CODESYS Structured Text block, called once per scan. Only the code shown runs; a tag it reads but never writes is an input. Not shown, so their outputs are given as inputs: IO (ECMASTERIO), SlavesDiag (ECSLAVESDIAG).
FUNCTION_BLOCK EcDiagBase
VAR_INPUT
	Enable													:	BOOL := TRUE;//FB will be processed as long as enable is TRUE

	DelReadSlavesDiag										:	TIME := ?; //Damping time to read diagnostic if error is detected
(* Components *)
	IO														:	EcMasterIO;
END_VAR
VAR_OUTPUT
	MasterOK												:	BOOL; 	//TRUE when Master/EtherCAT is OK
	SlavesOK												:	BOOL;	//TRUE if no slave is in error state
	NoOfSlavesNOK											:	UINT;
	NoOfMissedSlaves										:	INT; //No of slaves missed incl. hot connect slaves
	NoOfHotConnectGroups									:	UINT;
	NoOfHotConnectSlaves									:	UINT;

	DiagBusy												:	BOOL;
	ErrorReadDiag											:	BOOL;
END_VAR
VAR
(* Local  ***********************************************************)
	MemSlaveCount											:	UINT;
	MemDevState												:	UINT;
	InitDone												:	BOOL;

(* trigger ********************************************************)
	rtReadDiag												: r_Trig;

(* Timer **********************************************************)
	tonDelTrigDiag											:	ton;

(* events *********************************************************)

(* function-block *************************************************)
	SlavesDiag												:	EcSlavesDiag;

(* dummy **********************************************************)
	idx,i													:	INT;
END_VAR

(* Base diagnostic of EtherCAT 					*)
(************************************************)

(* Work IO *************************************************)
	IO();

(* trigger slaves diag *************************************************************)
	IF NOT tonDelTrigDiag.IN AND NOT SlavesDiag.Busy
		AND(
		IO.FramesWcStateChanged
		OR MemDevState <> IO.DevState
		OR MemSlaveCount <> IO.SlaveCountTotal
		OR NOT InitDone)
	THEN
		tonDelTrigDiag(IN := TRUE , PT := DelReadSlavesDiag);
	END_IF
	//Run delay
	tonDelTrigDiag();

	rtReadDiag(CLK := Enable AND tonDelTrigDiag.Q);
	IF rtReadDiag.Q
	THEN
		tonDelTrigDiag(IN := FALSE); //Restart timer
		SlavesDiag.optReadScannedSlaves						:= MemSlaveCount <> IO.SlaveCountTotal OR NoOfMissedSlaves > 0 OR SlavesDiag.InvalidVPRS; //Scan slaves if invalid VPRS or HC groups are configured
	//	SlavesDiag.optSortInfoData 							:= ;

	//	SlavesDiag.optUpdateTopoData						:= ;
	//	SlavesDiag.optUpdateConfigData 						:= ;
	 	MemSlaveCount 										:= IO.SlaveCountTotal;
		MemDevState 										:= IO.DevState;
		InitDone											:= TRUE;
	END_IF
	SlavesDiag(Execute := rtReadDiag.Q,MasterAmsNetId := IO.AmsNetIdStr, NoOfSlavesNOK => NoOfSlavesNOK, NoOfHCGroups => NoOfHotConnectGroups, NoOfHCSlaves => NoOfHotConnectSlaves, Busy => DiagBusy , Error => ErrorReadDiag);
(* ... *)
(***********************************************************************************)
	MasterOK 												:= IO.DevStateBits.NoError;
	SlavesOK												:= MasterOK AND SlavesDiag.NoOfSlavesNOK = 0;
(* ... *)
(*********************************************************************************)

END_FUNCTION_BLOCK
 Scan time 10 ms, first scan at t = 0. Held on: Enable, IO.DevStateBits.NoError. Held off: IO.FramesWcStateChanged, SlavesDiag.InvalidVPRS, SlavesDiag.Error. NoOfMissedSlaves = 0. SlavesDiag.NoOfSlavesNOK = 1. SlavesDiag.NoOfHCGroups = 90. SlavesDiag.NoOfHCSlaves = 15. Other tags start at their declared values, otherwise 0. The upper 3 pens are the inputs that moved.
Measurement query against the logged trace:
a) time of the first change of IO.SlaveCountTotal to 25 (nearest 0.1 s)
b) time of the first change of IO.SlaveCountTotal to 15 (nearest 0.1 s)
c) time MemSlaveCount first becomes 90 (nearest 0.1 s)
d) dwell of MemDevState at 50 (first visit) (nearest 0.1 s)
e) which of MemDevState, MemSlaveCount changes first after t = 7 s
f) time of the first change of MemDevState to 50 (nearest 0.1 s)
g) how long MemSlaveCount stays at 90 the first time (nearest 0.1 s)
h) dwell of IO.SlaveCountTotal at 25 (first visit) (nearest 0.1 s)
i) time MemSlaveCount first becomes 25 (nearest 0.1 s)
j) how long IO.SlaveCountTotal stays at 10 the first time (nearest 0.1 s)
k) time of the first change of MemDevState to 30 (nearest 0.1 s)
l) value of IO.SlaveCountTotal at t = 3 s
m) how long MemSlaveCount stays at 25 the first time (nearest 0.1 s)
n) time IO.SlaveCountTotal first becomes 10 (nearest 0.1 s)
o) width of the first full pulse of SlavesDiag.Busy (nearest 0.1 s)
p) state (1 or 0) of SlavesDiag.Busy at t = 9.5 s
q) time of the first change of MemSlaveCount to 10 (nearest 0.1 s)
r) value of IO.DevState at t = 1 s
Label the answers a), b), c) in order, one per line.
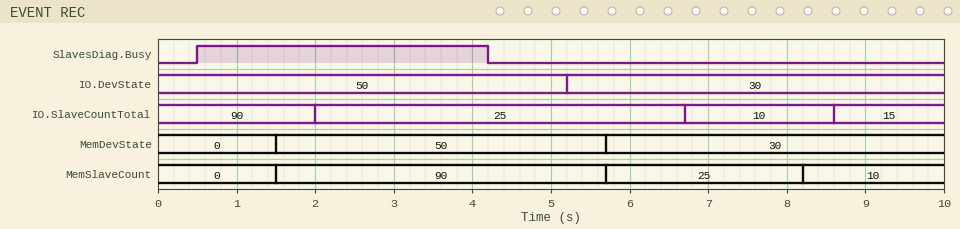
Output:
a) 2.0 s
b) 8.6 s
c) 1.5 s
d) 4.2 s
e) MemSlaveCount
f) 1.5 s
g) 4.2 s
h) 4.7 s
i) 5.7 s
j) 1.9 s
k) 5.7 s
l) 25
m) 2.5 s
n) 6.7 s
o) 3.7 s
p) 0
q) 8.2 s
r) 50
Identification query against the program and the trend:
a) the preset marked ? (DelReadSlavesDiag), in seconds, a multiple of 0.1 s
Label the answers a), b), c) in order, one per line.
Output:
a) 1.5 s
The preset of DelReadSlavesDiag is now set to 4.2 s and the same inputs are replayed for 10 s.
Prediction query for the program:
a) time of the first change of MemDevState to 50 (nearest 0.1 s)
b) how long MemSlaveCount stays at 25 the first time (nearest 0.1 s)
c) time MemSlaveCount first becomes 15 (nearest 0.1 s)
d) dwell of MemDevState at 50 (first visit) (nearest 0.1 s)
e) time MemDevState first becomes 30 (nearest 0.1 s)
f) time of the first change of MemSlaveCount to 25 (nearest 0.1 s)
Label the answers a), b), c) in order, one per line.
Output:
a) 4.2 s
b) 5.2 s
c) 9.4 s
d) 5.2 s
e) 9.4 s
f) 4.2 s
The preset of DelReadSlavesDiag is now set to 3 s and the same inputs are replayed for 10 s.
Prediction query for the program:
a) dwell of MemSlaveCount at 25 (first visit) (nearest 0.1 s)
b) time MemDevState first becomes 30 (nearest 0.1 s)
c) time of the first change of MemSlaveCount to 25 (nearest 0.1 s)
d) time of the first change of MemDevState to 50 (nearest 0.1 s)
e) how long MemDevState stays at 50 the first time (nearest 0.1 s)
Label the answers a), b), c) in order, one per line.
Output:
a) 5.2 s
b) 8.2 s
c) 3.0 s
d) 3.0 s
e) 5.2 s
